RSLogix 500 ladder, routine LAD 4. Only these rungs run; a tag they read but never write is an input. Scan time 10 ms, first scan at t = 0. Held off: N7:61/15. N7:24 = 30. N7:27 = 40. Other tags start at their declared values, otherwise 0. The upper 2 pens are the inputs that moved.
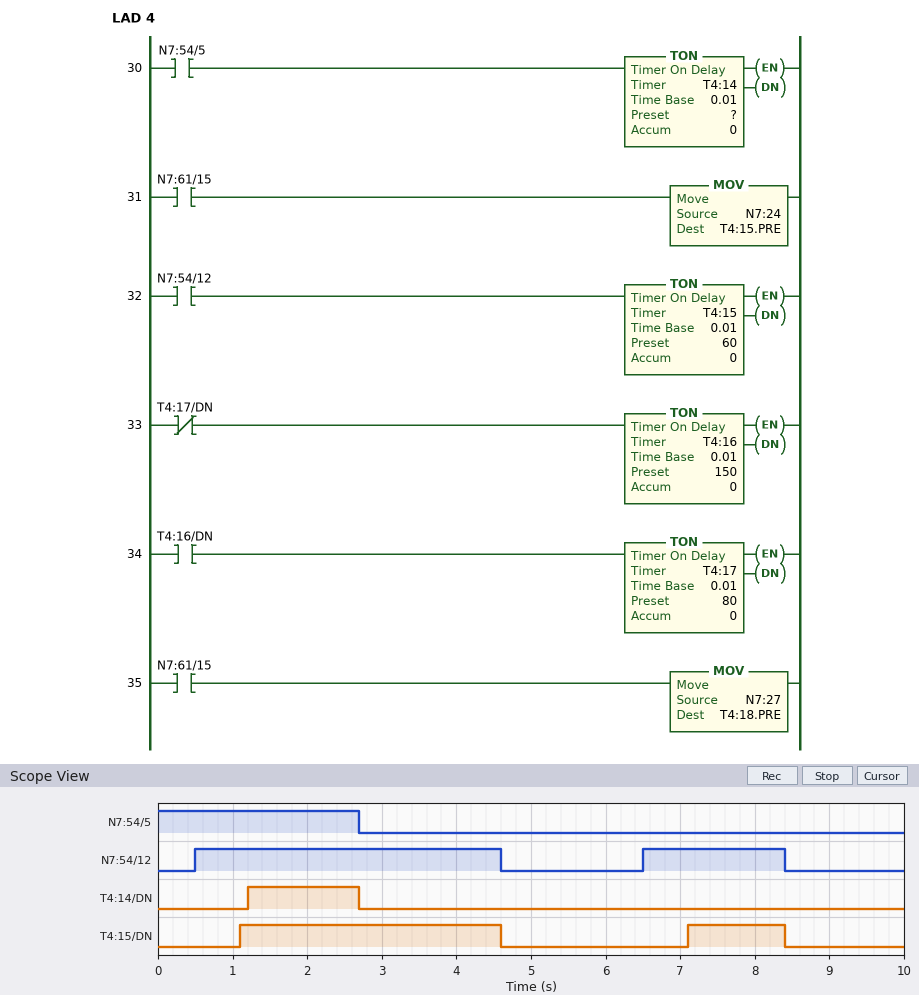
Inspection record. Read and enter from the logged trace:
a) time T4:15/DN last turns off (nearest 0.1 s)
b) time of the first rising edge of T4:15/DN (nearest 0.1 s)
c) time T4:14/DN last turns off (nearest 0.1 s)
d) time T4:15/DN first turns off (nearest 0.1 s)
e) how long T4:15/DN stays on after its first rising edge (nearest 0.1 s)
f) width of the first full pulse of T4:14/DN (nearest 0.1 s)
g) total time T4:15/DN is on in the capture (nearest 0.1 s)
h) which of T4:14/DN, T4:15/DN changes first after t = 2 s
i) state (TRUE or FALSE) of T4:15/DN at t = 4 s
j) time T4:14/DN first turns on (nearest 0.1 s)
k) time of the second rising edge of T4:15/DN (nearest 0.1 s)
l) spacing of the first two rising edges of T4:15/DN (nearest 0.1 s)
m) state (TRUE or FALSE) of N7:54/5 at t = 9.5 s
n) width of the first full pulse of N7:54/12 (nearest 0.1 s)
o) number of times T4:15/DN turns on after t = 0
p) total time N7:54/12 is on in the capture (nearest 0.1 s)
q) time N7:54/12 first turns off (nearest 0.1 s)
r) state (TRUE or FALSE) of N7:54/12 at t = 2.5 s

8.4 s
1.1 s
2.7 s
4.6 s
3.5 s
1.5 s
4.8 s
T4:14/DN
TRUE
1.2 s
7.1 s
6.0 s
FALSE
4.1 s
2
6.0 s
4.6 s
TRUE
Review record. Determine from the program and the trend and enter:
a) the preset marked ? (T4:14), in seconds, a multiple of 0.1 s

1.2 s
